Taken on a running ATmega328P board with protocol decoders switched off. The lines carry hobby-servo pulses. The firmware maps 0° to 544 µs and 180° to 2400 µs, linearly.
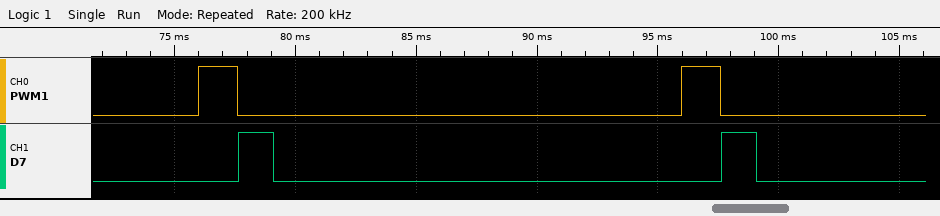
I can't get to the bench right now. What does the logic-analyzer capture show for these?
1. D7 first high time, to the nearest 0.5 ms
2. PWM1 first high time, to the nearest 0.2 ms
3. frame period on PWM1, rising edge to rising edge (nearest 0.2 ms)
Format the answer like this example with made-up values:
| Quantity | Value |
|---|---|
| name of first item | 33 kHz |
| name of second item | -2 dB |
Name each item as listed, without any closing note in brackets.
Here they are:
| Quantity | Value |
|---|---|
| D7 first high time, to the nearest 0.5 ms | 1.5 ms |
| PWM1 first high time, to the nearest 0.2 ms | 1.6 ms |
| frame period on PWM1, rising edge to rising edge | 20.0 ms |
